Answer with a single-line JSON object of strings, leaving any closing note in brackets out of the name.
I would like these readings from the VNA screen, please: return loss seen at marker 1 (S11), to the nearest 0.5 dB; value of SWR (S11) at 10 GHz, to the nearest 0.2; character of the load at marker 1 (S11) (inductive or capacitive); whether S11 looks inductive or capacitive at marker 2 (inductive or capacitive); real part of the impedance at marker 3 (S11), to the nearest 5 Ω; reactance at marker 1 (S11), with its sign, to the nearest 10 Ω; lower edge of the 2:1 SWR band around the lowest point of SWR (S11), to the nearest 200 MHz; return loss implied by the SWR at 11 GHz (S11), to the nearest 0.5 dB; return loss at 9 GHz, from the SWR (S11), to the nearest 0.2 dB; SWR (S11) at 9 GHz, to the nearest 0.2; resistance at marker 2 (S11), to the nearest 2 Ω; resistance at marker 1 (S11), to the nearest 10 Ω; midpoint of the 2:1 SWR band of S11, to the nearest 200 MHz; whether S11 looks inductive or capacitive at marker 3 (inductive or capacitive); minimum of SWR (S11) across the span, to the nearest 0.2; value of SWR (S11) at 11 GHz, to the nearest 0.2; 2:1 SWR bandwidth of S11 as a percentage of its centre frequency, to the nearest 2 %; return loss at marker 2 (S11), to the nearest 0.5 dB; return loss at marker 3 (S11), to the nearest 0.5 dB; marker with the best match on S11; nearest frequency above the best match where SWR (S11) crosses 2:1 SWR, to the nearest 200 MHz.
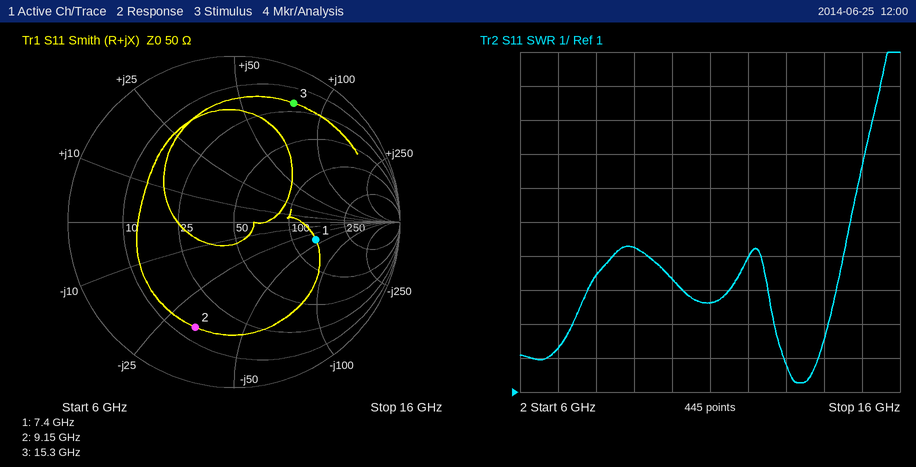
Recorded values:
{"return loss seen at marker 1 (S11), to the nearest 0.5 dB": "6.0 dB", "value of SWR (S11) at 10 GHz, to the nearest 0.2": "4.4", "character of the load at marker 1 (S11)": "capacitive", "whether S11 looks inductive or capacitive at marker 2": "capacitive", "real part of the impedance at marker 3 (S11), to the nearest 5 Ω": "20 Ω", "reactance at marker 1 (S11), with its sign, to the nearest 10 Ω": "-40 Ω", "lower edge of the 2:1 SWR band around the lowest point of SWR (S11), to the nearest 200 MHz": "13.0 GHz", "return loss implied by the SWR at 11 GHz (S11), to the nearest 0.5 dB": "5.0 dB", "return loss at 9 GHz, from the SWR (S11), to the nearest 0.2 dB": "3.4 dB", "SWR (S11) at 9 GHz, to the nearest 0.2": "5.2", "resistance at marker 2 (S11), to the nearest 2 Ω": "14 Ω", "resistance at marker 1 (S11), to the nearest 10 Ω": "140 Ω", "midpoint of the 2:1 SWR band of S11, to the nearest 200 MHz": "13.4 GHz", "whether S11 looks inductive or capacitive at marker 3": "inductive", "minimum of SWR (S11) across the span, to the nearest 0.2": "1.2", "value of SWR (S11) at 11 GHz, to the nearest 0.2": "3.6", "2:1 SWR bandwidth of S11 as a percentage of its centre frequency, to the nearest 2 %": "6 %", "return loss at marker 2 (S11), to the nearest 0.5 dB": "3.5 dB", "return loss at marker 3 (S11), to the nearest 0.5 dB": "2.0 dB", "marker with the best match on S11": "marker 1", "nearest frequency above the best match where SWR (S11) crosses 2:1 SWR, to the nearest 200 MHz": "13.8 GHz"}
